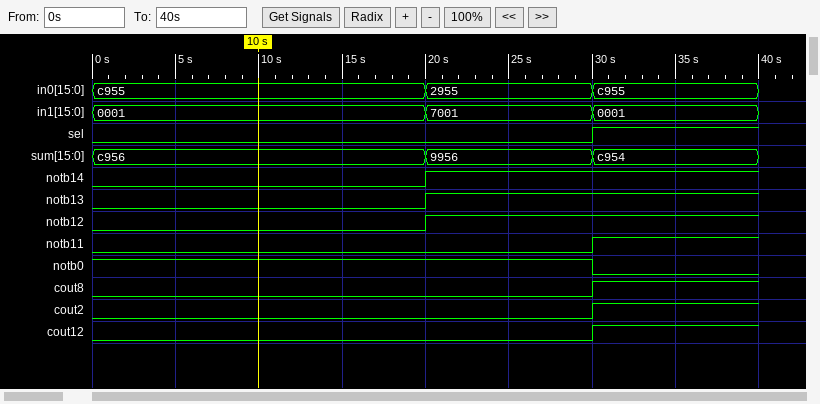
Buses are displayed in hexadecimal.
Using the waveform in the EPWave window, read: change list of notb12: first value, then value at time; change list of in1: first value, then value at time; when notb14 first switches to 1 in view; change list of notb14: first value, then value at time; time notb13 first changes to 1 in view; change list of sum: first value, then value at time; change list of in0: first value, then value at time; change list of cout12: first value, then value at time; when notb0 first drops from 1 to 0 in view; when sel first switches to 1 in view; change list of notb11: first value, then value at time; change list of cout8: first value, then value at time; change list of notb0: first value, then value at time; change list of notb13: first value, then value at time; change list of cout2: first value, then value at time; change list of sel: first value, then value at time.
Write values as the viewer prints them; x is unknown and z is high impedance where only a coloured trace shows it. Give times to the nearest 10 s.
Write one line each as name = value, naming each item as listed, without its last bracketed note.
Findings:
change list of notb12: first value, then value at time = 0, 1 at 20 s
change list of in1: first value, then value at time = 0001, 7001 at 20 s, 0001 at 30 s
when notb14 first switches to 1 in view = 20 s
change list of notb14: first value, then value at time = 0, 1 at 20 s
time notb13 first changes to 1 in view = 20 s
change list of sum: first value, then value at time = c956, 9956 at 20 s, c954 at 30 s
change list of in0: first value, then value at time = c955, 2955 at 20 s, c955 at 30 s
change list of cout12: first value, then value at time = 0, 1 at 30 s
when notb0 first drops from 1 to 0 in view = 30 s
when sel first switches to 1 in view = 30 s
change list of notb11: first value, then value at time = 0, 1 at 30 s
change list of cout8: first value, then value at time = 0, 1 at 30 s
change list of notb0: first value, then value at time = 1, 0 at 30 s
change list of notb13: first value, then value at time = 0, 1 at 20 s
change list of cout2: first value, then value at time = 0, 1 at 30 s
change list of sel: first value, then value at time = 0, 1 at 30 s
